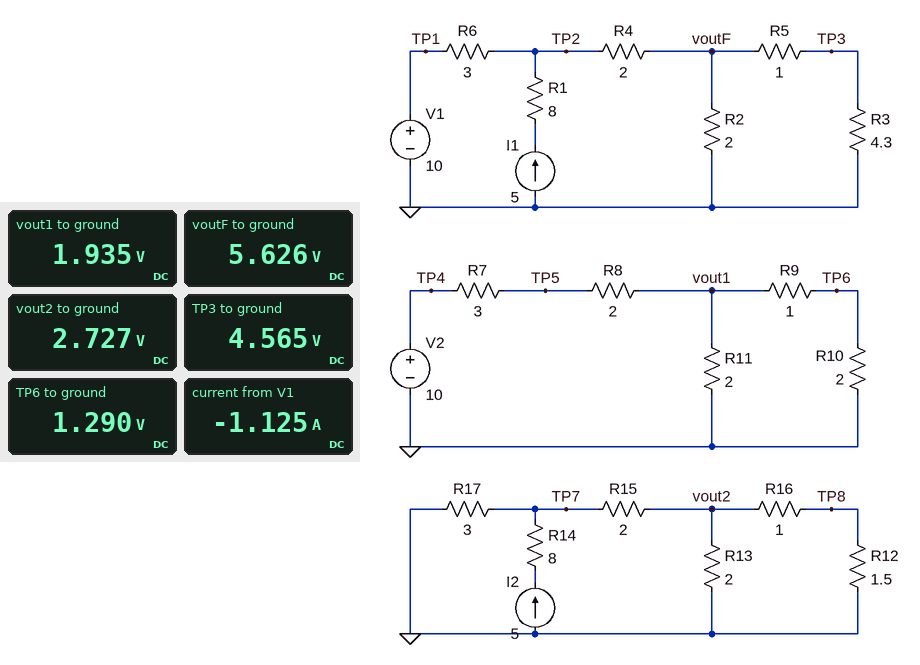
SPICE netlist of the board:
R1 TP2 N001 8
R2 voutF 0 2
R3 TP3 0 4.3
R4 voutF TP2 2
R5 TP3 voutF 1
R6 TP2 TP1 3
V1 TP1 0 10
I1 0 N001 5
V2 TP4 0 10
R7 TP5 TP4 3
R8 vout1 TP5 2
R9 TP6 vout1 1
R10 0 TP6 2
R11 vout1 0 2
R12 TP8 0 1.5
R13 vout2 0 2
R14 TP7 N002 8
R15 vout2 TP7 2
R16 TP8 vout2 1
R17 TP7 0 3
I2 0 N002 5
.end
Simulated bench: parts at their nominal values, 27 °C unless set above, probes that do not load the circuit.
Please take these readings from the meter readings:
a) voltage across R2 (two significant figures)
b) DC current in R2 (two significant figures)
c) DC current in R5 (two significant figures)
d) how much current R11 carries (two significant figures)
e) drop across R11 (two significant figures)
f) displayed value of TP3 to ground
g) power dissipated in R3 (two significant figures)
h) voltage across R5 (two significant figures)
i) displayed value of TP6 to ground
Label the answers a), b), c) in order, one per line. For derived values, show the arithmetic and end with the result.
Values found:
a) 5.626 V = 5.6 V
b) (5.626 V) / 2 Ω = 2.8 A
c) (5.626 V - 4.565 V) / 1 Ω = 1.1 A
d) (1.935 V) / 2 Ω = 970 mA
e) 1.935 V = 1.9 V
f) 4.565 V
g) (4.565 V)^2 / 4.3 Ω = 4.8 W
h) 5.626 V - 4.565 V = 1.1 V
i) 1.290 V
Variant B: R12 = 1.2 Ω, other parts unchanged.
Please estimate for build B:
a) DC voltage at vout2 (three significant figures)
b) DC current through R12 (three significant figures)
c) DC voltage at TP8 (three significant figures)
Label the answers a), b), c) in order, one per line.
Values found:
a) 2.60 V
b) 1.18 A
c) 1.42 V
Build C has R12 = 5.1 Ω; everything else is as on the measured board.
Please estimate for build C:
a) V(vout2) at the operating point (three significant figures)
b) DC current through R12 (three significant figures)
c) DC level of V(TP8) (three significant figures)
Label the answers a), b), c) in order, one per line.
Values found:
a) 3.47 V
b) 569 mA
c) 2.90 V
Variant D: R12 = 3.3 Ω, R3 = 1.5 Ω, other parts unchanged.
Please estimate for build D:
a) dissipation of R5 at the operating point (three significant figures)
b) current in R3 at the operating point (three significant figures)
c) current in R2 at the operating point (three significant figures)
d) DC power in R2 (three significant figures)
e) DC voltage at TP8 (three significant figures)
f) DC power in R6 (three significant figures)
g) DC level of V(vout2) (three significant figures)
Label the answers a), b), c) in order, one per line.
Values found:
a) 3.31 W
b) 1.82 A
c) 2.27 A
d) 10.3 W
e) 2.47 V
f) 2.48 W
g) 3.22 V
